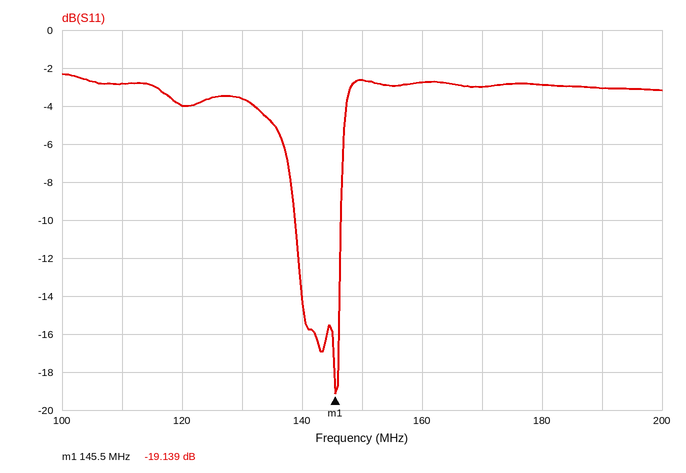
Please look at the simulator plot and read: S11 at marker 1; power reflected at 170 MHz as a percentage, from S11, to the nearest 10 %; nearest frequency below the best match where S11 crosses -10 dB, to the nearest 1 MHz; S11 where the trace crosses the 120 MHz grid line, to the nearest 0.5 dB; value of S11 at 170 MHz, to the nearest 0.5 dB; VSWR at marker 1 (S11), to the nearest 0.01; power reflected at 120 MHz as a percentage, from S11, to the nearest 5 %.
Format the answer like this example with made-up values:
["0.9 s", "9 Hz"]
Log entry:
["-19.139 dB", "50 %", "139 MHz", "-4.0 dB", "-3.0 dB", "1.25", "40 %"]
